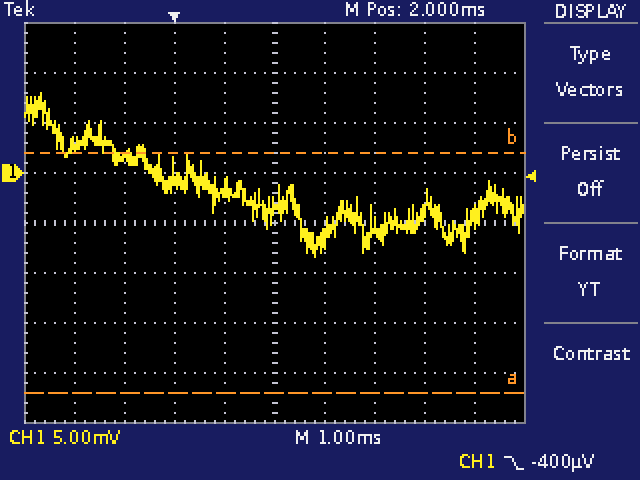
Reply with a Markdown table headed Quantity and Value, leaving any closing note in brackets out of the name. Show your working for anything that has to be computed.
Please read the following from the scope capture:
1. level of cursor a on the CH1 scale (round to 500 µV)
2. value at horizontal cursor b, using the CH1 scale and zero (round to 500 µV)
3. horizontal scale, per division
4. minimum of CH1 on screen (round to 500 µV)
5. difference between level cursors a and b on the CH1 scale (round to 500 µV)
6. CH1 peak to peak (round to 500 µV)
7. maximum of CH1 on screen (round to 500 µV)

| Quantity | Value |
|---|---|
| level of cursor a on the CH1 scale | -22.0 mV |
| value at horizontal cursor b, using the CH1 scale and zero | 2.0 mV |
| horizontal scale, per division | 1 ms |
| minimum of CH1 on screen | -8.5 mV |
| difference between level cursors a and b on the CH1 scale | 24.0 mV |
| CH1 peak to peak | 8.0 mV − (-8.5 mV) = 16.5 mV |
| maximum of CH1 on screen | 8.0 mV |
